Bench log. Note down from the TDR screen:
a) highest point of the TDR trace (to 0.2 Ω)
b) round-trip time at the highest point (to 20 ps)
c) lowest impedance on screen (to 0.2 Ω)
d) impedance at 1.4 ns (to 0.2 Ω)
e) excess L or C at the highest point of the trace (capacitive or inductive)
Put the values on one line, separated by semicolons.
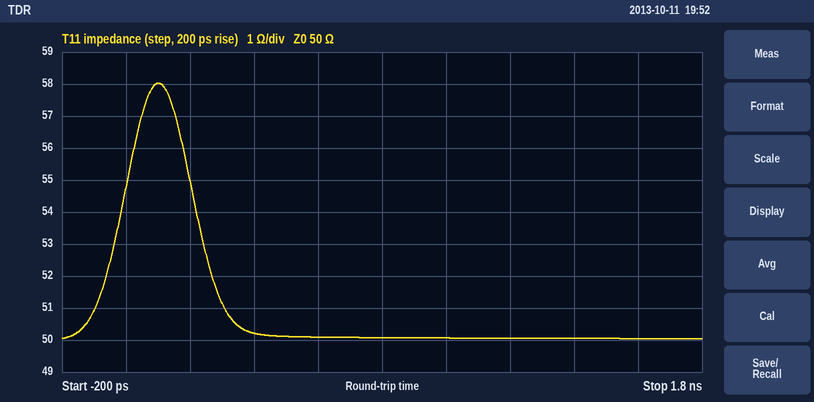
58.0 Ω; 100 ps; 50.0 Ω; 50.0 Ω; inductive
